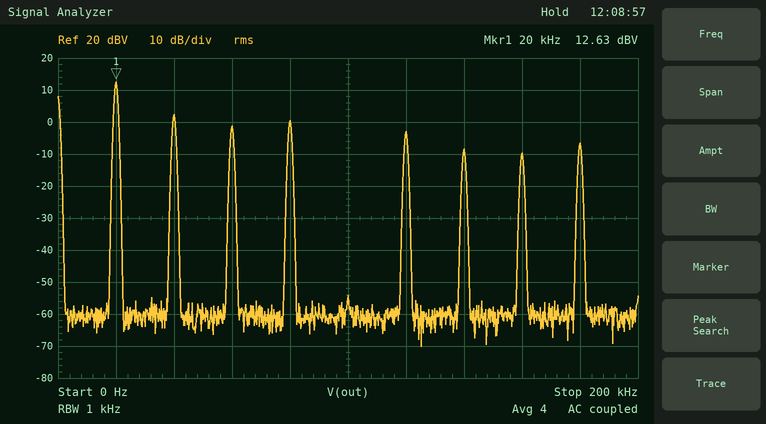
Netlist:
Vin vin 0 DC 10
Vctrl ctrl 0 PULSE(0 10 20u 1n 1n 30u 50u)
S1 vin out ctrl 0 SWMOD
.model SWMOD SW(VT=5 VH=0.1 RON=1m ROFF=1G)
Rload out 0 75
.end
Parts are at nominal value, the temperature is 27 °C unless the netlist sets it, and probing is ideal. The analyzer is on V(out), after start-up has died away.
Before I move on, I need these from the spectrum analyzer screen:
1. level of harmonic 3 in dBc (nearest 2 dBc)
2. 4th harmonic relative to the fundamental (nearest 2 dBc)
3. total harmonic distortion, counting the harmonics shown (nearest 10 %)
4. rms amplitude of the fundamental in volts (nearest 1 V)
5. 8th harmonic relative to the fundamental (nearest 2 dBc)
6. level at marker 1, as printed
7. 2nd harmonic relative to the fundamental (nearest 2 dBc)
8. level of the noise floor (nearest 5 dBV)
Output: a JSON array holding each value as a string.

["-14 dBc", "-12 dBc", "50 %", "4 V", "-22 dBc", "12.63 dBV", "-10 dBc", "-60 dBV"]
